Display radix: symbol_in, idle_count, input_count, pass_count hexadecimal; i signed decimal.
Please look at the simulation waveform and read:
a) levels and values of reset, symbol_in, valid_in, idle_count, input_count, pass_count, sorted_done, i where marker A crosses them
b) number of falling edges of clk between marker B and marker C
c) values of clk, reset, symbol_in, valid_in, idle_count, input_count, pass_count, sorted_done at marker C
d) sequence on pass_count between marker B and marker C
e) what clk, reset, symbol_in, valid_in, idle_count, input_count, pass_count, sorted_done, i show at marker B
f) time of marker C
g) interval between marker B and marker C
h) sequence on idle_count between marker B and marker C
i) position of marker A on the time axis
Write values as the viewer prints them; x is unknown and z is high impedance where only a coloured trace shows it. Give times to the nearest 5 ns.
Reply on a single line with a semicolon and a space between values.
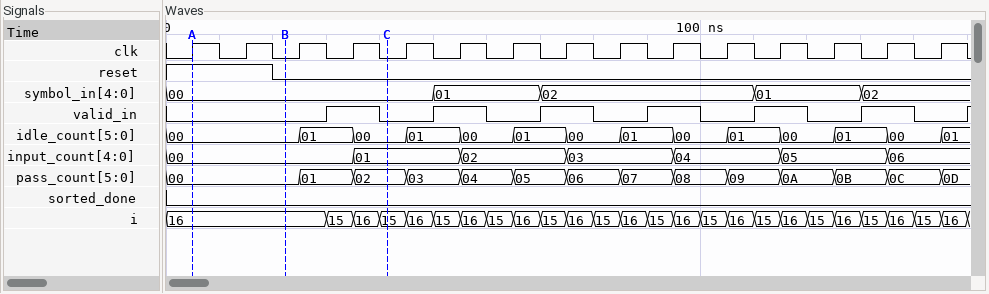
reset=1, symbol_in=00, valid_in=0, idle_count=00, input_count=00, pass_count=00, sorted_done=0, i=16; 2; clk=0, reset=0, symbol_in=00, valid_in=0, idle_count=00, input_count=01, pass_count=02, sorted_done=0; 00, 01, 02; clk=0, reset=0, symbol_in=00, valid_in=0, idle_count=00, input_count=00, pass_count=00, sorted_done=0, i=16; 40 ns; 20 ns; 00, 01, 00; 5 ns
